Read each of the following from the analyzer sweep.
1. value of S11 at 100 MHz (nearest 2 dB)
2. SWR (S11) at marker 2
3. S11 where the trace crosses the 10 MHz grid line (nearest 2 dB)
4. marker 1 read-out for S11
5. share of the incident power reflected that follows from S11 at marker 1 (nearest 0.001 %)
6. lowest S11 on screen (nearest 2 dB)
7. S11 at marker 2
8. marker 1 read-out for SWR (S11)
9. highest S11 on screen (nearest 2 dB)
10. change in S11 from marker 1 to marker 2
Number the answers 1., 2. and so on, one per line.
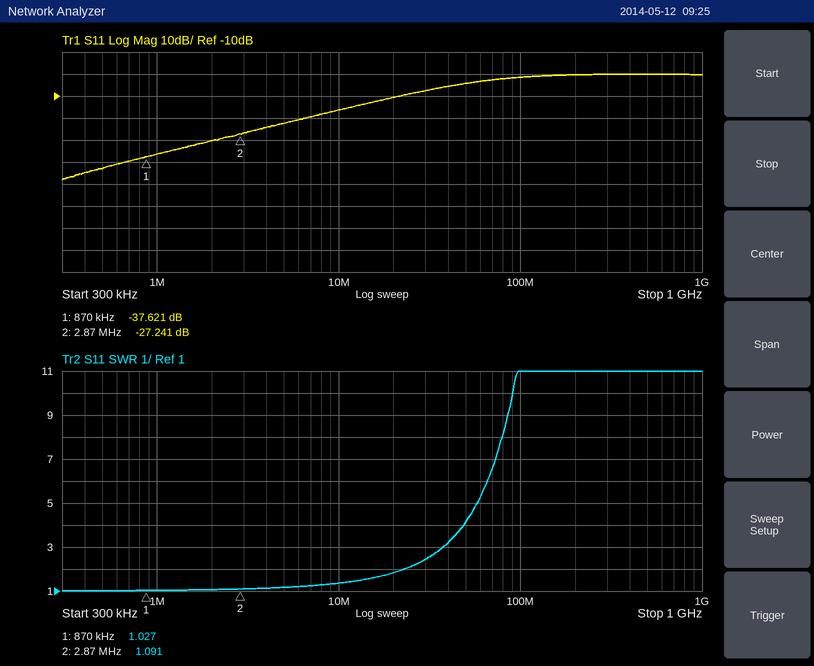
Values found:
1. -2 dB
2. 1.091
3. -16 dB
4. -37.621 dB
5. 0.017 %
6. -48 dB
7. -27.241 dB
8. 1.027
9. 0 dB
10. 10.380 dB
